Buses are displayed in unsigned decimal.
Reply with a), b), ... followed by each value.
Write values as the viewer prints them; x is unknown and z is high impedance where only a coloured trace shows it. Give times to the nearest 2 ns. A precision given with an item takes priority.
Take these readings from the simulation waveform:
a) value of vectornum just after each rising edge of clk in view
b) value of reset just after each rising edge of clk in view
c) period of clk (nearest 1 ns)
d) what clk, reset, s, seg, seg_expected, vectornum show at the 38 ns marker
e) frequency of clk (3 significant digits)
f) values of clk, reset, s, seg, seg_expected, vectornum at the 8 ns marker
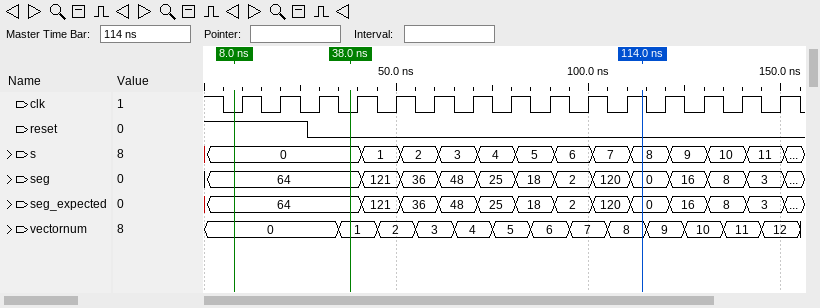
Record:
a) 0, 0, 0, 1, 2, 3, 4, 5, 6, 7, 8, 9, 10, 11, 12
b) 1 1 0 0 0 0 0 0 0 0 0 0 0 0 0
c) 10 ns
d) clk=0, reset=0, s=0, seg=64, seg_expected=64, vectornum=1
e) 100 MHz
f) clk=0, reset=1, s=0, seg=64, seg_expected=64, vectornum=0
